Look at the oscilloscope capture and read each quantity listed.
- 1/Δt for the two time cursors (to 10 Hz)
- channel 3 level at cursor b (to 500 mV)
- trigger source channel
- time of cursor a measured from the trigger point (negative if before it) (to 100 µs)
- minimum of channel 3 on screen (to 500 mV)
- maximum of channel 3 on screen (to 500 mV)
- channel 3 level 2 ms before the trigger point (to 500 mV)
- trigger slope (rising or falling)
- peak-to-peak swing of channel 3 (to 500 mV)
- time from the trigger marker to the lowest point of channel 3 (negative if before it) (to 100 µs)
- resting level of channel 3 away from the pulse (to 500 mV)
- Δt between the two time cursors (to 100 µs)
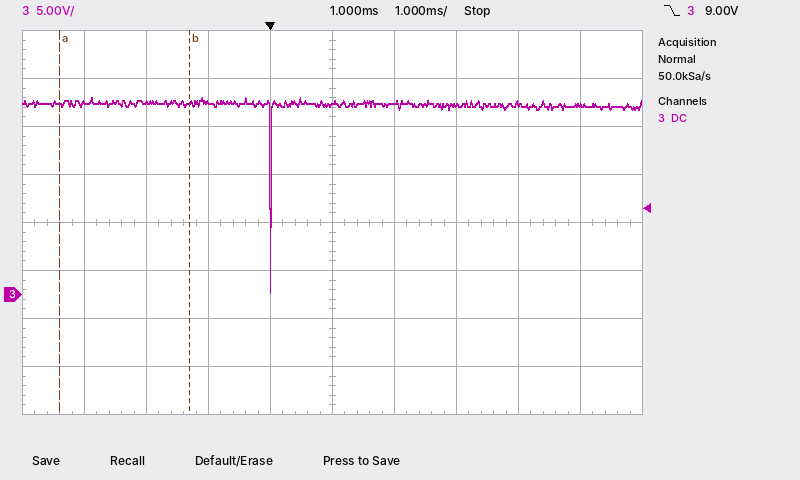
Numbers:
480 Hz
20.0 V
channel 3
-3.4 ms
0.0 V
20.5 V
20.0 V
falling
20.5 V
0.0 ms
20.0 V
2.1 ms
